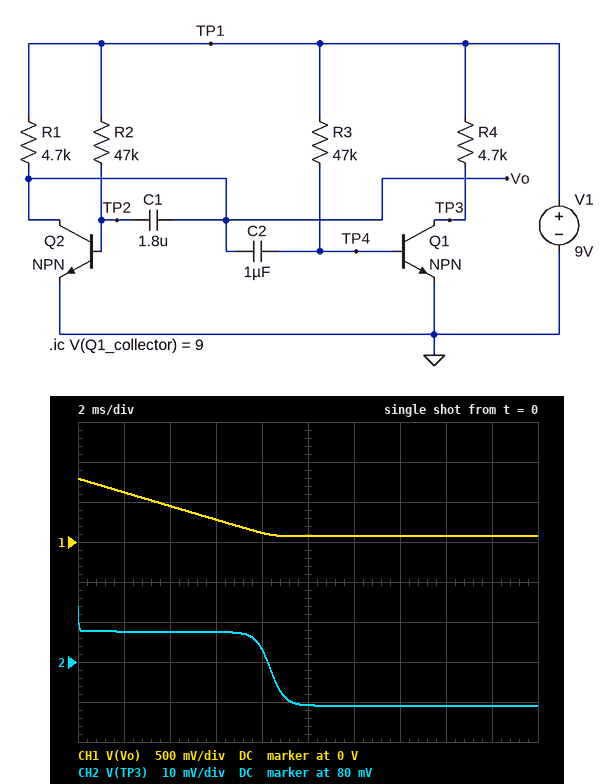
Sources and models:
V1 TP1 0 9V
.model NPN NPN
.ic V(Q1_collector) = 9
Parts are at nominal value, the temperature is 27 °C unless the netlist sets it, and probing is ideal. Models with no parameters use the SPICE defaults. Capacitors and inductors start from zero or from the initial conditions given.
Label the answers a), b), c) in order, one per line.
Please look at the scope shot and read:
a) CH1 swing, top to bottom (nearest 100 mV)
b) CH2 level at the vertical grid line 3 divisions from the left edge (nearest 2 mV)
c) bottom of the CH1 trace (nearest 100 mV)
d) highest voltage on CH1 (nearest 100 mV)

a) 700 mV
b) 88 mV
c) 100 mV
d) 800 mV
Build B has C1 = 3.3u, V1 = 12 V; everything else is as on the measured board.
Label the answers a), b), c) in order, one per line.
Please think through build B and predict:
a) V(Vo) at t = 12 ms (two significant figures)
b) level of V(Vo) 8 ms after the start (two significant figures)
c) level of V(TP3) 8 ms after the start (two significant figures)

a) 75 mV
b) 290 mV
c) 77 mV
